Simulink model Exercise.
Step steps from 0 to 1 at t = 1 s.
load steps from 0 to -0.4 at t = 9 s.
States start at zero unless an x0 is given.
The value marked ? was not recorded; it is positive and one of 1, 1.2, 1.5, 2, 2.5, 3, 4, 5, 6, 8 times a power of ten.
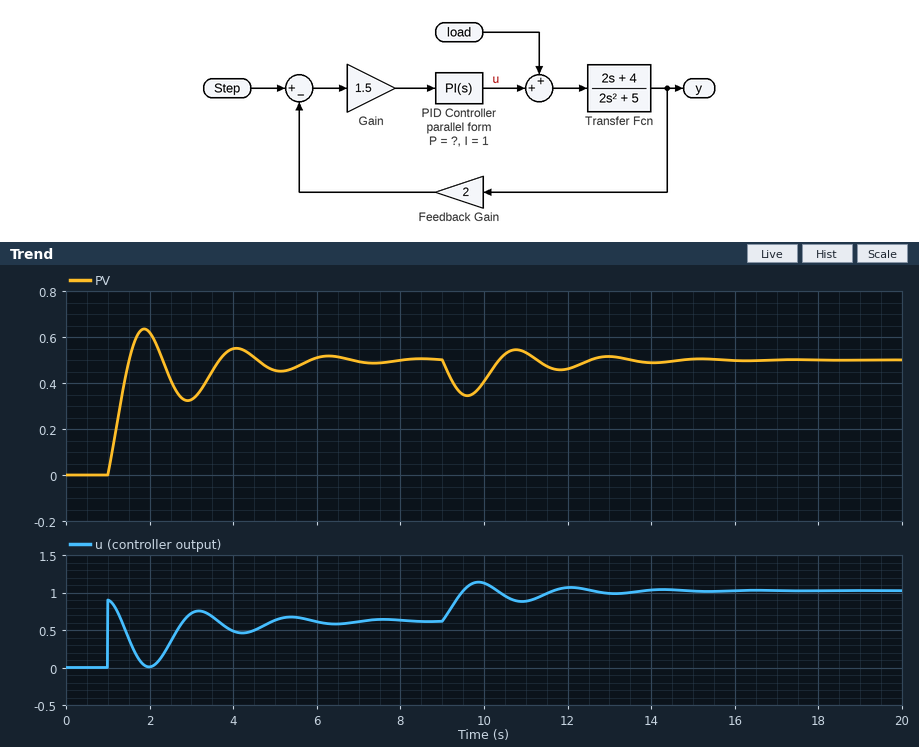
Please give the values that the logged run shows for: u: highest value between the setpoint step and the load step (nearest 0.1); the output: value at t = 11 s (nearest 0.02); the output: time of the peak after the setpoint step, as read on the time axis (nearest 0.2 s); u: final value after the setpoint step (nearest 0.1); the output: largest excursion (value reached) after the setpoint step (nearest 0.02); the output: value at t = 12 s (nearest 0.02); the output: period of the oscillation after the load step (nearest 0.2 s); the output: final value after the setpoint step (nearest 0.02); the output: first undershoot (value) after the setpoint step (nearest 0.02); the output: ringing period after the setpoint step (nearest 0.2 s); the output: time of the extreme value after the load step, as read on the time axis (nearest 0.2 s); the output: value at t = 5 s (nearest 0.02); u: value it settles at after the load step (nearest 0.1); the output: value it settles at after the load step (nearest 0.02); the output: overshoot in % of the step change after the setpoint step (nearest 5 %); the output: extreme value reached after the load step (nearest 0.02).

0.9
0.54
1.8 s
0.6
0.64
0.46
2.2 s
0.50
0.32
2.2 s
9.6 s
0.46
1.0
0.50
25 %
0.34
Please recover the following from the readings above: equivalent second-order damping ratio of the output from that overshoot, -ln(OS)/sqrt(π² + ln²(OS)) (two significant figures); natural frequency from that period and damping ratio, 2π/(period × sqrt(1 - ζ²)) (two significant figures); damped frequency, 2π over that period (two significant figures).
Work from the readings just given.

0.40
3.1 rad/s
2.9 rad/s
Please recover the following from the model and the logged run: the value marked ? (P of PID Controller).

0.6
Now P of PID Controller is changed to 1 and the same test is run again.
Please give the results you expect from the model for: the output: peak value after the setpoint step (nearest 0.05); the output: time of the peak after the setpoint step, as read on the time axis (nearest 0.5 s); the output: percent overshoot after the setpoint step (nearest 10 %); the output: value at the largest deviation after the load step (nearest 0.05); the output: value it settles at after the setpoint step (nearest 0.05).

0.60
1.5 s
20 %
0.40
0.50
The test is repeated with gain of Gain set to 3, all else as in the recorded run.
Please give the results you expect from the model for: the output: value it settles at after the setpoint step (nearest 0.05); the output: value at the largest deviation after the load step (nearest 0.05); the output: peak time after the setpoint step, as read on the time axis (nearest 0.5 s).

0.50
0.40
1.5 s
